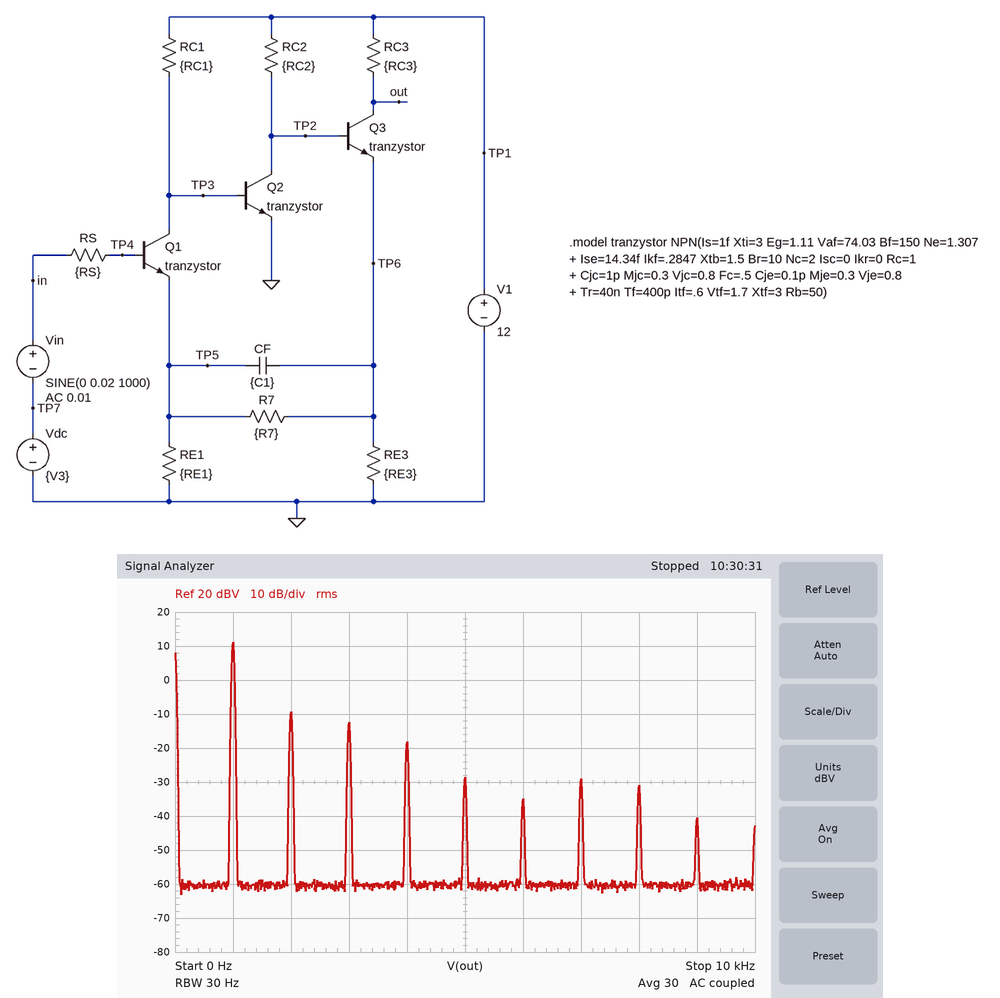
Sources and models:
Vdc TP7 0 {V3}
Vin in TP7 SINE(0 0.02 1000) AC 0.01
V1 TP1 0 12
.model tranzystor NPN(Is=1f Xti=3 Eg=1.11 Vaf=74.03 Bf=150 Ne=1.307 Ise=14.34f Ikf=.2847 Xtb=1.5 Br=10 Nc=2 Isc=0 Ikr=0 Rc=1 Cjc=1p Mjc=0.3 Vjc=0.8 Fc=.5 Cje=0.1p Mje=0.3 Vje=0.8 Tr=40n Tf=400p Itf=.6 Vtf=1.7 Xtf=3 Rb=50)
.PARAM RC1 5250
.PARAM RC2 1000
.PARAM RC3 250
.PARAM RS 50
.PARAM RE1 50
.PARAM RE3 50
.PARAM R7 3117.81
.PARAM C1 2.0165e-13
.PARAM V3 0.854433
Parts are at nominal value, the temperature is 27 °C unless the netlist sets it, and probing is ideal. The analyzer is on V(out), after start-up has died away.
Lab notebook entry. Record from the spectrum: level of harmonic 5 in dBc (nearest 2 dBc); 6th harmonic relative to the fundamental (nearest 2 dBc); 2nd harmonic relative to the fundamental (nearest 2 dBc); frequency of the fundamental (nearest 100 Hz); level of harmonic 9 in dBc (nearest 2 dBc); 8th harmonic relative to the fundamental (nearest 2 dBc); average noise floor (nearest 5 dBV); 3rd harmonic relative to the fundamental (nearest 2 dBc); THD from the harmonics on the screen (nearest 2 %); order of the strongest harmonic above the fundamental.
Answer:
-40 dBc
-46 dBc
-20 dBc
1.0 kHz
-52 dBc
-42 dBc
-60 dBV
-24 dBc
12 %
2
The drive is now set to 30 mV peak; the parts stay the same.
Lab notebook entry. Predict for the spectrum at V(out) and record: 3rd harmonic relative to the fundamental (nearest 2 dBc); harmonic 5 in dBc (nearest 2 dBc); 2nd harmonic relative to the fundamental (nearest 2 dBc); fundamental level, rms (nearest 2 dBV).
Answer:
-14 dBc
-38 dBc
-18 dBc
12 dBV
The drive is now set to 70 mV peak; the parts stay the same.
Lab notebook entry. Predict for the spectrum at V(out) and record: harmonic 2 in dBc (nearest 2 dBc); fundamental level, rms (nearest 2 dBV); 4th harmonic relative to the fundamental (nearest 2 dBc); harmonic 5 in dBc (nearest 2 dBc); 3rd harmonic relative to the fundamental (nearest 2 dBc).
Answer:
-24 dBc
12 dBV
-26 dBc
-16 dBc
-10 dBc
